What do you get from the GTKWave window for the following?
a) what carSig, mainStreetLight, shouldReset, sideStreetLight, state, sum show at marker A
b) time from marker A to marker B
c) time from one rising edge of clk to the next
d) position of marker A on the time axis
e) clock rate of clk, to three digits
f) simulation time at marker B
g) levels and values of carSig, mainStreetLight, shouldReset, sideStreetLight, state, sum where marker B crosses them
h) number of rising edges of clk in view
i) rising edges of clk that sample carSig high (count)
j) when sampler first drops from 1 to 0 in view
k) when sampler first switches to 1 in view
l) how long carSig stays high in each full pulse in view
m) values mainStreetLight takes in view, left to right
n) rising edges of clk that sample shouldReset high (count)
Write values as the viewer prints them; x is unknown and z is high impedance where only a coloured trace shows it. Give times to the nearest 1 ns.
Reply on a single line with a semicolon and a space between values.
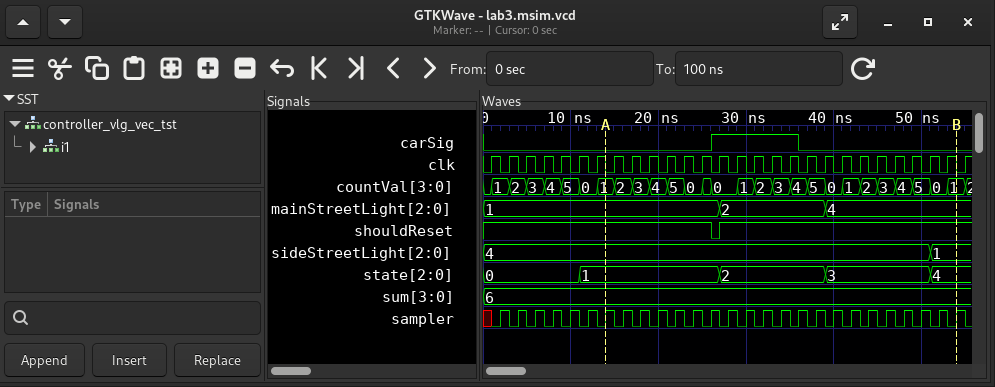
carSig=0, mainStreetLight=1, shouldReset=1, sideStreetLight=4, state=1, sum=6; 40 ns; 2 ns; 14 ns; 500 MHz; 54 ns; carSig=0, mainStreetLight=4, shouldReset=1, sideStreetLight=1, state=4, sum=6; 28; 5; 3 ns; 2 ns; 10 ns; 1, 2, 4; 27
